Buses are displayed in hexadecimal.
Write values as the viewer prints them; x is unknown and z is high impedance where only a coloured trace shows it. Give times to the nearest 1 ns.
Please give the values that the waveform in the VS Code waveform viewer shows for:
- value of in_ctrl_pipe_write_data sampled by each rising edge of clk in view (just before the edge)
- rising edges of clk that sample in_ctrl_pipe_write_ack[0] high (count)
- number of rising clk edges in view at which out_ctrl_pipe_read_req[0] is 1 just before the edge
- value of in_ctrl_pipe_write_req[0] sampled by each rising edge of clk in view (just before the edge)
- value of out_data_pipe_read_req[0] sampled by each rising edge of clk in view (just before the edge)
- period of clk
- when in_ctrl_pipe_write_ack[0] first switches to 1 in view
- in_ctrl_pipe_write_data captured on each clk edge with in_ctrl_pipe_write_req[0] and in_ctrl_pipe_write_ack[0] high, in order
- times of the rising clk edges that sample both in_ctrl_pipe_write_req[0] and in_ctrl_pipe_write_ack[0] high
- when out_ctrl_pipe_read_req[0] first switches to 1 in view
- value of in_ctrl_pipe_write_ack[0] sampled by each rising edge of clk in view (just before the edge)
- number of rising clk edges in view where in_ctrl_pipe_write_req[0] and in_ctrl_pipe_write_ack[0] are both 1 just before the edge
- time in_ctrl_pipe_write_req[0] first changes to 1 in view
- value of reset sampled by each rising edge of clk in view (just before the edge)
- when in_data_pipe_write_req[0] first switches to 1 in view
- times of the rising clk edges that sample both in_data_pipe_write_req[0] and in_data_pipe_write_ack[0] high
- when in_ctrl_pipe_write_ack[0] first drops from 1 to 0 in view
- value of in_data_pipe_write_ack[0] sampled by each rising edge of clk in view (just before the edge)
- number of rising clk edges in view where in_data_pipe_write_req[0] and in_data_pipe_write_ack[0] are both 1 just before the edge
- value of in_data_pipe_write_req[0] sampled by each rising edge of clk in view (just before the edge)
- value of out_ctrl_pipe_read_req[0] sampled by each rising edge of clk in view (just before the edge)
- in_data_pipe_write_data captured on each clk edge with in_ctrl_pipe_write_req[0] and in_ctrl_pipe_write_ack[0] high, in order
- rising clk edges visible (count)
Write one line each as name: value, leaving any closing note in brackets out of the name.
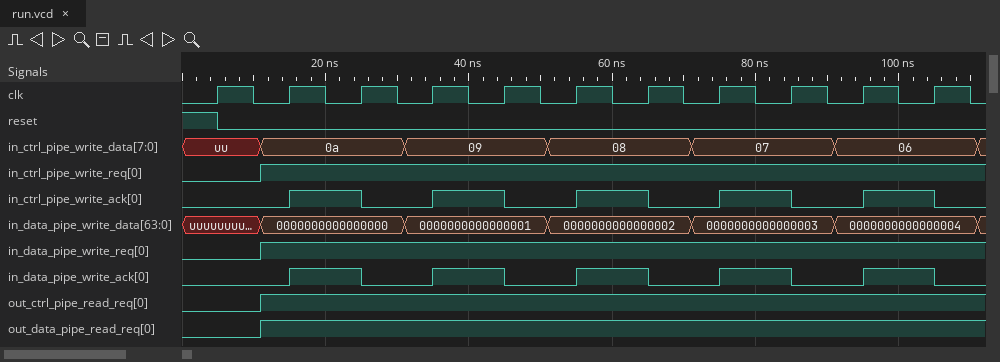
value of in_ctrl_pipe_write_data sampled by each rising edge of clk in view: uu, 0a, 0a, 09, 09, 08, 08, 07, 07, 06, 06
rising edges of clk that sample in_ctrl_pipe_write_ack[0] high: 5
number of rising clk edges in view at which out_ctrl_pipe_read_req[0] is 1 just before the edge: 10
value of in_ctrl_pipe_write_req[0] sampled by each rising edge of clk in view: 0 1 1 1 1 1 1 1 1 1 1
value of out_data_pipe_read_req[0] sampled by each rising edge of clk in view: 0 1 1 1 1 1 1 1 1 1 1
period of clk: 10 ns
when in_ctrl_pipe_write_ack[0] first switches to 1 in view: 15 ns
in_ctrl_pipe_write_data captured on each clk edge with in_ctrl_pipe_write_req[0] and in_ctrl_pipe_write_ack[0] high, in order: 0a, 09, 08, 07, 06
times of the rising clk edges that sample both in_ctrl_pipe_write_req[0] and in_ctrl_pipe_write_ack[0] high: 25 ns, 45 ns, 65 ns, 85 ns, 105 ns
when out_ctrl_pipe_read_req[0] first switches to 1 in view: 11 ns
value of in_ctrl_pipe_write_ack[0] sampled by each rising edge of clk in view: 0 0 1 0 1 0 1 0 1 0 1
number of rising clk edges in view where in_ctrl_pipe_write_req[0] and in_ctrl_pipe_write_ack[0] are both 1 just before the edge: 5
time in_ctrl_pipe_write_req[0] first changes to 1 in view: 11 ns
value of reset sampled by each rising edge of clk in view: 1 0 0 0 0 0 0 0 0 0 0
when in_data_pipe_write_req[0] first switches to 1 in view: 11 ns
times of the rising clk edges that sample both in_data_pipe_write_req[0] and in_data_pipe_write_ack[0] high: 25 ns, 45 ns, 65 ns, 85 ns, 105 ns
when in_ctrl_pipe_write_ack[0] first drops from 1 to 0 in view: 25 ns
value of in_data_pipe_write_ack[0] sampled by each rising edge of clk in view: 0 0 1 0 1 0 1 0 1 0 1
number of rising clk edges in view where in_data_pipe_write_req[0] and in_data_pipe_write_ack[0] are both 1 just before the edge: 5
value of in_data_pipe_write_req[0] sampled by each rising edge of clk in view: 0 1 1 1 1 1 1 1 1 1 1
value of out_ctrl_pipe_read_req[0] sampled by each rising edge of clk in view: 0 1 1 1 1 1 1 1 1 1 1
in_data_pipe_write_data captured on each clk edge with in_ctrl_pipe_write_req[0] and in_ctrl_pipe_write_ack[0] high, in order: 0000000000000000, 0000000000000001, 0000000000000002, 0000000000000003, 0000000000000004
rising clk edges visible: 11
